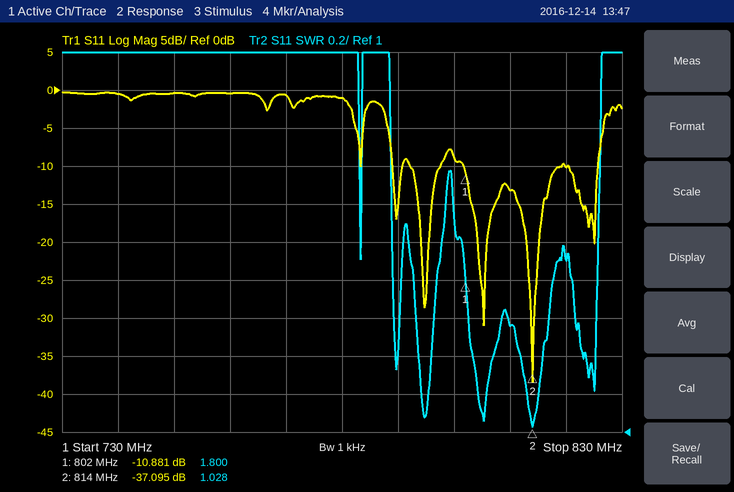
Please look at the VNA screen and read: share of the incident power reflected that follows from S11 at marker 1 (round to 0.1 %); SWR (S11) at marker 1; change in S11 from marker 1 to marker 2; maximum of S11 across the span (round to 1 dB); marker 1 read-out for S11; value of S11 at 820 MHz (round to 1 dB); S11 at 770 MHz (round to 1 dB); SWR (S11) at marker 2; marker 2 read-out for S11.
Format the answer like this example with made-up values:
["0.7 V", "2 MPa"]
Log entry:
["8.2 %", "1.800", "-26.214 dB", "0 dB", "-10.881 dB", "-10 dB", "-1 dB", "1.028", "-37.095 dB"]
